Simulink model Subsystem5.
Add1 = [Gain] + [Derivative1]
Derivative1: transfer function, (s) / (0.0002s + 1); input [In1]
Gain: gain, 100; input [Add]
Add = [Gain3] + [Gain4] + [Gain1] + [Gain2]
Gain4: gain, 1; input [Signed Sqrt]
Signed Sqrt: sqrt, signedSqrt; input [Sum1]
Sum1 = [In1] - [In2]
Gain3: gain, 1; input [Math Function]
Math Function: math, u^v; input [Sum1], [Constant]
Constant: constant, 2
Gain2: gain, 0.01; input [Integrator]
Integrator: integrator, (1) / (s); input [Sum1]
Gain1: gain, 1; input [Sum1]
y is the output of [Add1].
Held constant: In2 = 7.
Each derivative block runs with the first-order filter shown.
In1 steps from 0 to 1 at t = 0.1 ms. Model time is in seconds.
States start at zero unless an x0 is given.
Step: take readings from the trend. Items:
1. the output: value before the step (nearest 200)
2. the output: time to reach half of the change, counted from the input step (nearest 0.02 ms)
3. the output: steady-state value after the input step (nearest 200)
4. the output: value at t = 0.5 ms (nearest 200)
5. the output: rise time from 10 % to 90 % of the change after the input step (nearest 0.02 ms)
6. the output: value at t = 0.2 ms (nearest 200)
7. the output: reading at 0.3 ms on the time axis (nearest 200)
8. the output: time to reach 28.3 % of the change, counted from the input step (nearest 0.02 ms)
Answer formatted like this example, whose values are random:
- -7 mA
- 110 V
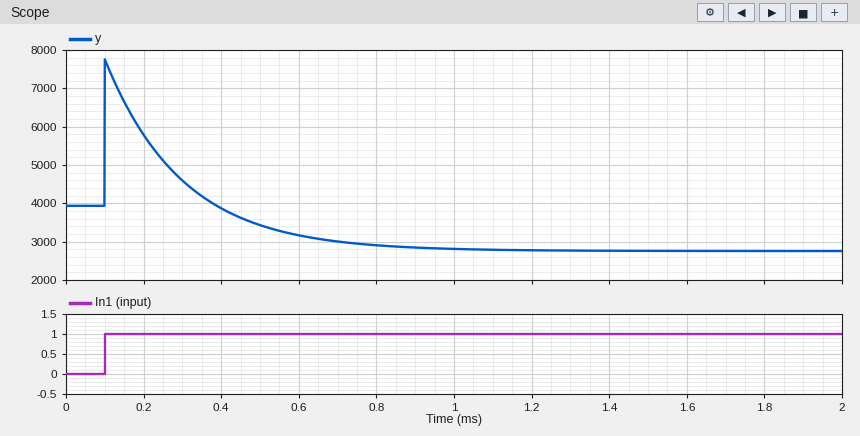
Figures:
- 4000
- 0.42 ms
- 2800
- 3400
- 0.44 ms
- 5800
- 4600
- 0.36 ms
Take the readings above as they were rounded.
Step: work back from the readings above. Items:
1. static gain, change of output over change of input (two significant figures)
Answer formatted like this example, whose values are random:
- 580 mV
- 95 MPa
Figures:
- -1200
